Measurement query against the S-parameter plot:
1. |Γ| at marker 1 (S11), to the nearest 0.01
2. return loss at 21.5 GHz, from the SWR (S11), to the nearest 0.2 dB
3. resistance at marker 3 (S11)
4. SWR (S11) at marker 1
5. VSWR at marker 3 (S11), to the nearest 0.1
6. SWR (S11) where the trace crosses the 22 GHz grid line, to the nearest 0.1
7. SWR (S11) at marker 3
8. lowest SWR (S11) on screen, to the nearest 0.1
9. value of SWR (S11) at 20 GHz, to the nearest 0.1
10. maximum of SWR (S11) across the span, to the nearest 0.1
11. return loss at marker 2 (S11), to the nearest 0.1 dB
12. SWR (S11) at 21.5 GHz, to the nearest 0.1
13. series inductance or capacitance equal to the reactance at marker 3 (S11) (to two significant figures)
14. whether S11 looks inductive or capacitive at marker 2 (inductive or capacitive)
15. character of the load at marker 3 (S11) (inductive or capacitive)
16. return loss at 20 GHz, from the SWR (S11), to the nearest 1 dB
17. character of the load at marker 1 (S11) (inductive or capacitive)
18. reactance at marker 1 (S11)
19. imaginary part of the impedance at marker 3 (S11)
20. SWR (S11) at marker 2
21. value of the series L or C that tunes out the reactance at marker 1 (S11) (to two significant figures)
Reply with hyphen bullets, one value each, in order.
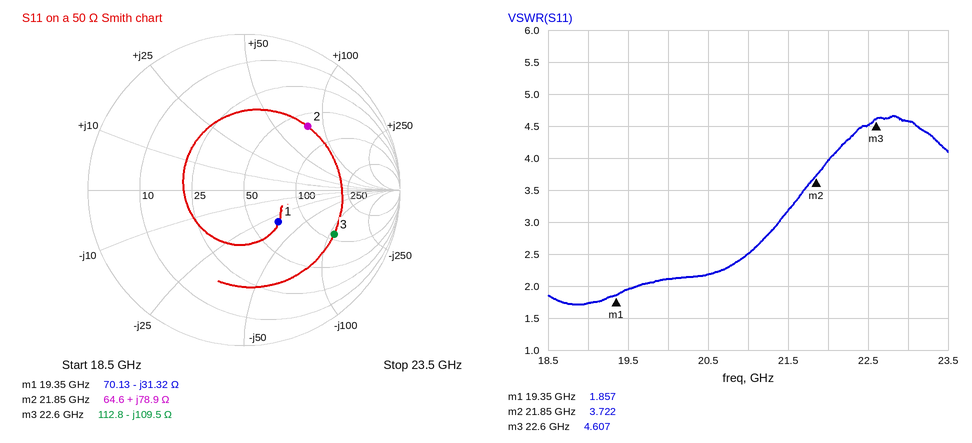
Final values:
- 0.30
- 5.6 dB
- 112.8 Ω
- 1.857
- 4.6
- 4.0
- 4.607
- 1.7
- 2.1
- 4.7
- 4.8 dB
- 3.2
- 64 fF
- inductive
- capacitive
- 9 dB
- capacitive
- -31.32 Ω
- -109.5 Ω
- 3.722
- 260 pH
